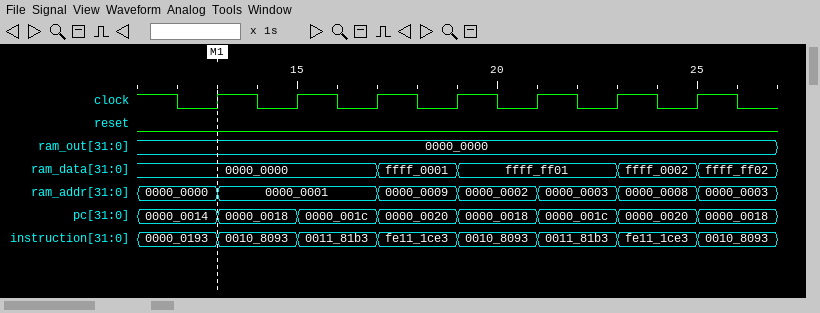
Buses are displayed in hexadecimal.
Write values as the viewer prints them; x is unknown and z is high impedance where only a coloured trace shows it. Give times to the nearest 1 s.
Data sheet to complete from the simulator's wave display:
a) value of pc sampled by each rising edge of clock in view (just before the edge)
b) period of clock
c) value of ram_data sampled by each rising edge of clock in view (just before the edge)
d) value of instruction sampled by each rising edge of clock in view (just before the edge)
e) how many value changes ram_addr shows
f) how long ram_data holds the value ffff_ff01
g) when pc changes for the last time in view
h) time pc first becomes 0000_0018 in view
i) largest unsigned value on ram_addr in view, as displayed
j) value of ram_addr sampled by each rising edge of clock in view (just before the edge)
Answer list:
0000_0014, 0000_0018, 0000_001c, 0000_0020, 0000_0018, 0000_001c, 0000_0020
2 s
0000_0000, 0000_0000, 0000_0000, ffff_0001, ffff_ff01, ffff_ff01, ffff_0002
0000_0193, 0010_8093, 0011_81b3, fe11_1ce3, 0010_8093, 0011_81b3, fe11_1ce3
6
4 s
25 s
13 s
0000_0009
0000_0000, 0000_0001, 0000_0001, 0000_0009, 0000_0002, 0000_0003, 0000_0008
